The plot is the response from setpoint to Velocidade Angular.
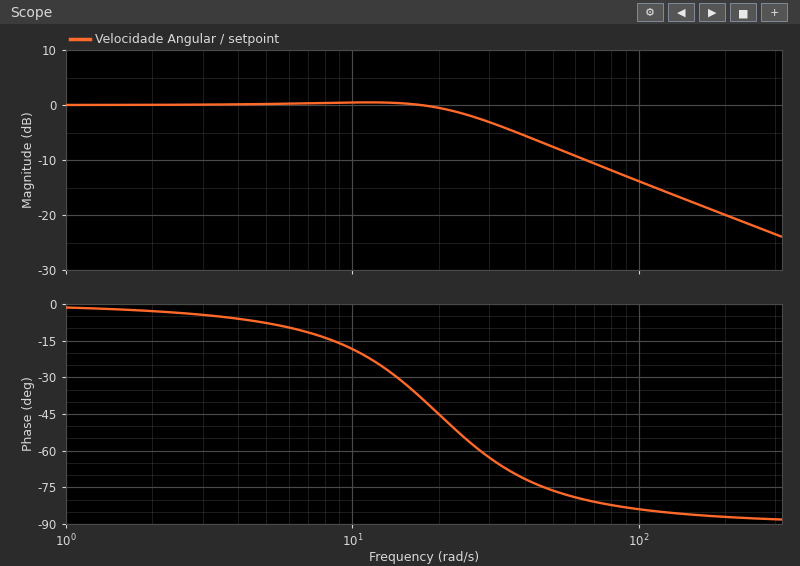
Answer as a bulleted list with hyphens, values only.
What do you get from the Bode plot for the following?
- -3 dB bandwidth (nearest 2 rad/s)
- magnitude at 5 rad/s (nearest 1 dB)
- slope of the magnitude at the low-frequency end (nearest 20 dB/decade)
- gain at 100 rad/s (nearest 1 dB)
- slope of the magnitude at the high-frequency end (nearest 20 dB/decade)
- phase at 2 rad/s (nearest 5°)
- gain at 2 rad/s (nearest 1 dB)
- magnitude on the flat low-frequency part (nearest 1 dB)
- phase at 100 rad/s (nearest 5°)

- 30 rad/s
- 0 dB
- 0 dB/decade
- -14 dB
- -20 dB/decade
- -5°
- 0 dB
- 0 dB
- -85°
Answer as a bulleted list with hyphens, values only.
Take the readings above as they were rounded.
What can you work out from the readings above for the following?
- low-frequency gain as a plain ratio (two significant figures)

- 1.0
